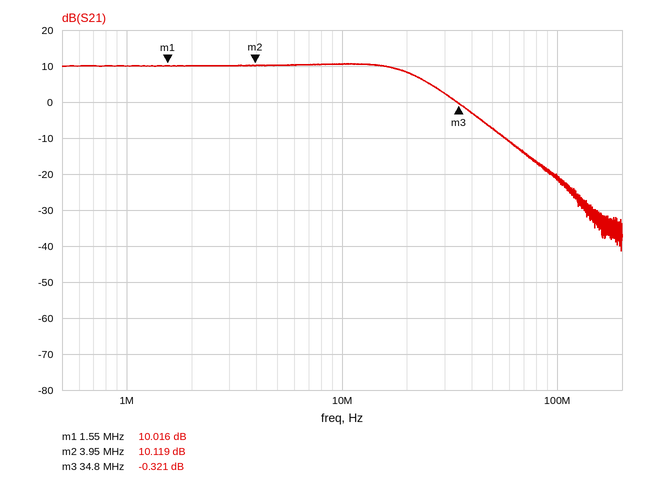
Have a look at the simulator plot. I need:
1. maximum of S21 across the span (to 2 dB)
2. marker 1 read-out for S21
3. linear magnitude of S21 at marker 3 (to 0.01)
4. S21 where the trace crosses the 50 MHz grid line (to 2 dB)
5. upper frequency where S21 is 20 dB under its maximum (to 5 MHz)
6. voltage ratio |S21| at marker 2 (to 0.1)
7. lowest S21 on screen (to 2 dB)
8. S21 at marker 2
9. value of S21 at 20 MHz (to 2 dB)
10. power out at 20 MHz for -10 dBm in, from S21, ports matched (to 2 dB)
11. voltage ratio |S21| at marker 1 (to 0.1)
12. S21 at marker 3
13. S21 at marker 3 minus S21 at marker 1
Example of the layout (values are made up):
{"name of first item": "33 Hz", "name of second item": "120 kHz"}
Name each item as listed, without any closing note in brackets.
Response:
{"maximum of S21 across the span": "10 dB", "marker 1 read-out for S21": "10.016 dB", "linear magnitude of S21 at marker 3": "0.96", "S21 where the trace crosses the 50 MHz grid line": "-8 dB", "upper frequency where S21 is 20 dB under its maximum": "55 MHz", "voltage ratio |S21| at marker 2": "3.2", "lowest S21 on screen": "-42 dB", "S21 at marker 2": "10.119 dB", "value of S21 at 20 MHz": "8 dB", "power out at 20 MHz for -10 dBm in, from S21, ports matched": "-2 dBm", "voltage ratio |S21| at marker 1": "3.2", "S21 at marker 3": "-0.321 dB", "S21 at marker 3 minus S21 at marker 1": "-10.337 dB"}
